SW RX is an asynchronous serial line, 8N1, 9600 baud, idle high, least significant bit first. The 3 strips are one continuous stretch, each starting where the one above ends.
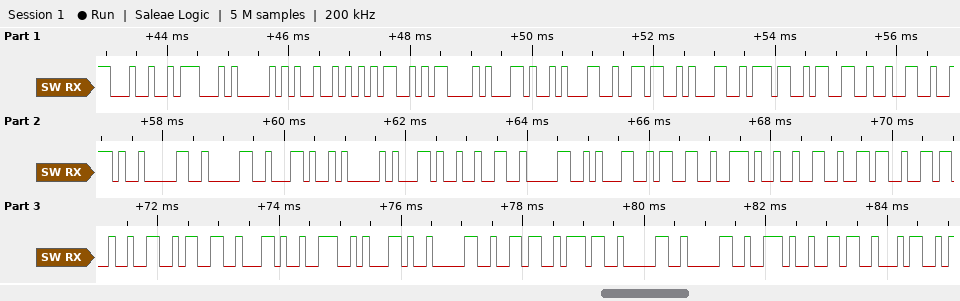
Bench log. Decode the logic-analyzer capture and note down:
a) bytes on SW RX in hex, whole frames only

0x24 0x47 0x50 0x52 0x4D 0x43 0x2C 0x31 0x36 0x31 0x37 0x33 0x32 0x2E 0x30 0x30 0x2C 0x41 0x2C 0x32 0x30 0x31 0x33 0x2E 0x32 0x36 0x36 0x32 0x33 0x2C 0x4E 0x2C 0x30 0x36 0x37 0x30 0x30 0x2E 0x36 0x34
